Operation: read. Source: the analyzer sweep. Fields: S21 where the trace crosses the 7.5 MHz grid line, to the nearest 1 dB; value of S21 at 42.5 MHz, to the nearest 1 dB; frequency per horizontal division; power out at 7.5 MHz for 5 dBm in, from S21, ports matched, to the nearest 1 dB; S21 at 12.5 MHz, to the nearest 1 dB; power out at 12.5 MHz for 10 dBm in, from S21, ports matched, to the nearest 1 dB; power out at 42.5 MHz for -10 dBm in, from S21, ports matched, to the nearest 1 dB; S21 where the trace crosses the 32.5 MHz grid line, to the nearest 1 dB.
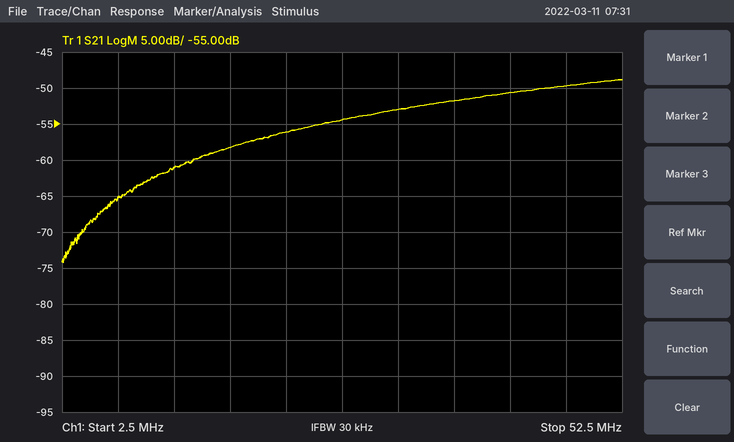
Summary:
-65 dB
-51 dB
5 MHz
-60 dBm
-61 dB
-51 dBm
-61 dBm
-53 dB
